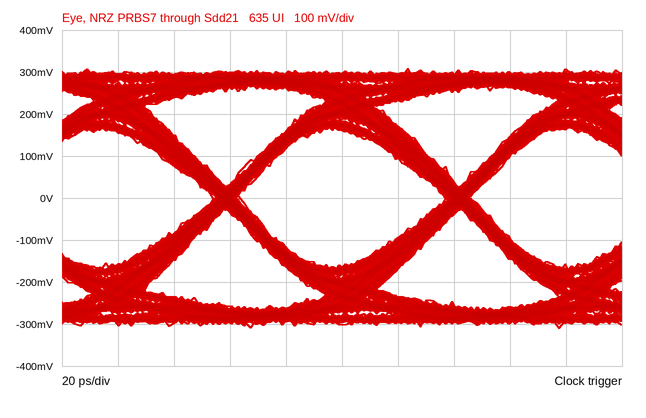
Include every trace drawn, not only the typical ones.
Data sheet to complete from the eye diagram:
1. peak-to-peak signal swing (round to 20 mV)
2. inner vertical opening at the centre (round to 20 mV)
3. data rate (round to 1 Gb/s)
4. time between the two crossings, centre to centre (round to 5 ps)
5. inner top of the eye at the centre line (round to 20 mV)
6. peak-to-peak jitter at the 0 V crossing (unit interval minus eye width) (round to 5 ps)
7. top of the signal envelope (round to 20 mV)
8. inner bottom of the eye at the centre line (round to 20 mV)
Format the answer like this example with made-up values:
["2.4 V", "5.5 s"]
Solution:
["620 mV", "320 mV", "12 Gb/s", "85 ps", "160 mV", "10 ps", "300 mV", "-160 mV"]
